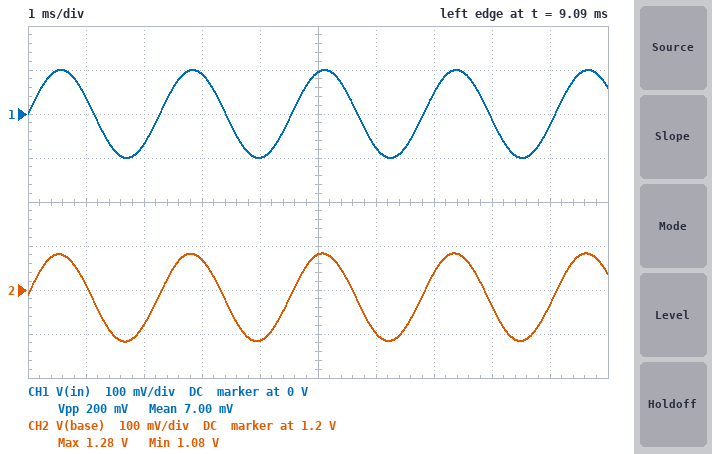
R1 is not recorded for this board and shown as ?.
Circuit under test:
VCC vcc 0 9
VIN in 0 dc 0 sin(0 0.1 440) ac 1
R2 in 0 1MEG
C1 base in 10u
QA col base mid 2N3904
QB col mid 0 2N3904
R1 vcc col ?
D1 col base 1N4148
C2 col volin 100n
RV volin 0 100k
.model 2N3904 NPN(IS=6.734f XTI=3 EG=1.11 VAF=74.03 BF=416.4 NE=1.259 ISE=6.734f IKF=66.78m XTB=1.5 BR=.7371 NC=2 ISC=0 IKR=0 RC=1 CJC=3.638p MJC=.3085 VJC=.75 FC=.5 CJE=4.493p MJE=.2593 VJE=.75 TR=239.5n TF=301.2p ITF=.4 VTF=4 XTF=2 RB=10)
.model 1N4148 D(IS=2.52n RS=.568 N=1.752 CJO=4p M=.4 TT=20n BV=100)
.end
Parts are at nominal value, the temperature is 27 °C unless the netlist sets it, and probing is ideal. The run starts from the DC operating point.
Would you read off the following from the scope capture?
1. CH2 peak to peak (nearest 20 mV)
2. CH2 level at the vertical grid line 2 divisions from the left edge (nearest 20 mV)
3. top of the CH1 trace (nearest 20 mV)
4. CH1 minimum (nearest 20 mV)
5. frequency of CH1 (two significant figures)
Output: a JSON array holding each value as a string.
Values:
["200 mV", "1.12 V", "100 mV", "-100 mV", "440 Hz"]
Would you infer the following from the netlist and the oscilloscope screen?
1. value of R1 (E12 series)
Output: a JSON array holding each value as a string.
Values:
["22 kΩ"]
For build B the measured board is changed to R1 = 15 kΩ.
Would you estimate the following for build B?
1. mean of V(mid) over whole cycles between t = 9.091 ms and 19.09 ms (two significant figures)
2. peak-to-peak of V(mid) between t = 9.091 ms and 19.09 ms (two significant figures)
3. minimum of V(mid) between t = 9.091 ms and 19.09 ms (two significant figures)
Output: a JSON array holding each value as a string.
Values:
["640 mV", "53 mV", "610 mV"]
